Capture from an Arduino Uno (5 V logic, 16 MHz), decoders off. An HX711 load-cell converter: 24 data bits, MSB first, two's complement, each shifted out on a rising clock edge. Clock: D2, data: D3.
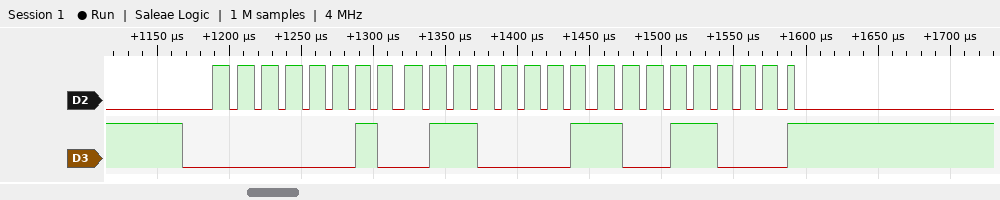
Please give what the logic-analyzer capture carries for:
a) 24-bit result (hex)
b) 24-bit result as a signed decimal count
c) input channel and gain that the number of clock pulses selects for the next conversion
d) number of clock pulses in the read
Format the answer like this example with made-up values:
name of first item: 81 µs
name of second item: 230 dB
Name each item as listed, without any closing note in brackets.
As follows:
24-bit result: 0x026198
24-bit result as a signed decimal count: 156056
input channel and gain that the number of clock pulses selects for the next conversion: channel A, gain 128
number of clock pulses in the read: 25
